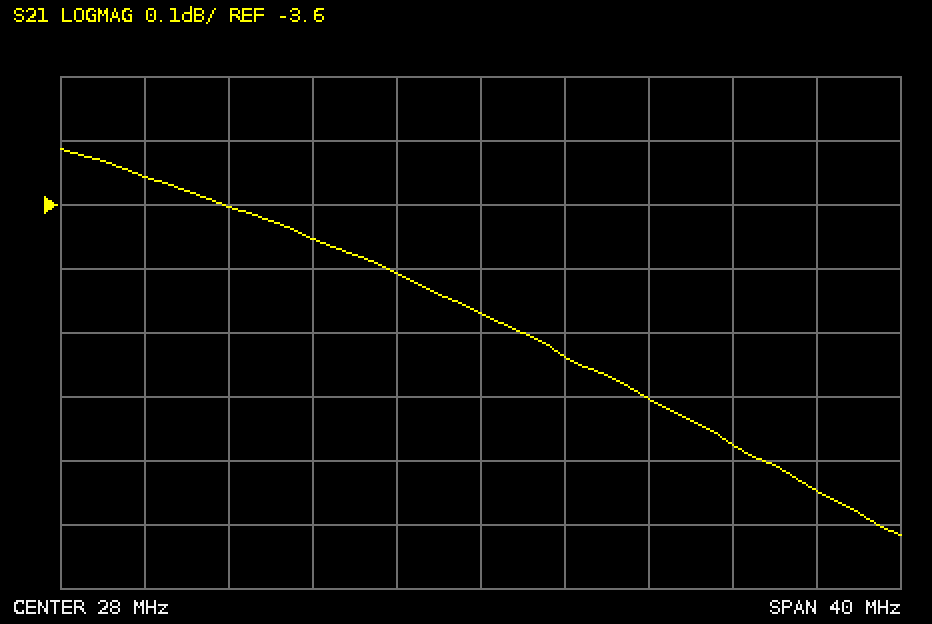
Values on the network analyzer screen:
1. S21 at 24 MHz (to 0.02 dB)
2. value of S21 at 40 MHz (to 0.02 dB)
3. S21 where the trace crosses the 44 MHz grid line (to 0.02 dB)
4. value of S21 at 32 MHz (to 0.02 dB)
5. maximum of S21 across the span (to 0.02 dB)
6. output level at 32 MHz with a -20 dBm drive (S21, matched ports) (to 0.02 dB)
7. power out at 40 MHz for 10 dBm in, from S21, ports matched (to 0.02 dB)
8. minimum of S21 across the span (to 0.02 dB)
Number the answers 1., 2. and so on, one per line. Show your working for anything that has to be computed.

1. -3.70 dB
2. -3.98 dB
3. -4.04 dB
4. -3.84 dB
5. -3.52 dB
6. -20 dBm + (-3.84 dB) = -23.84 dBm
7. 10 dBm + (-3.98 dB) = 6.02 dBm
8. -4.12 dB
